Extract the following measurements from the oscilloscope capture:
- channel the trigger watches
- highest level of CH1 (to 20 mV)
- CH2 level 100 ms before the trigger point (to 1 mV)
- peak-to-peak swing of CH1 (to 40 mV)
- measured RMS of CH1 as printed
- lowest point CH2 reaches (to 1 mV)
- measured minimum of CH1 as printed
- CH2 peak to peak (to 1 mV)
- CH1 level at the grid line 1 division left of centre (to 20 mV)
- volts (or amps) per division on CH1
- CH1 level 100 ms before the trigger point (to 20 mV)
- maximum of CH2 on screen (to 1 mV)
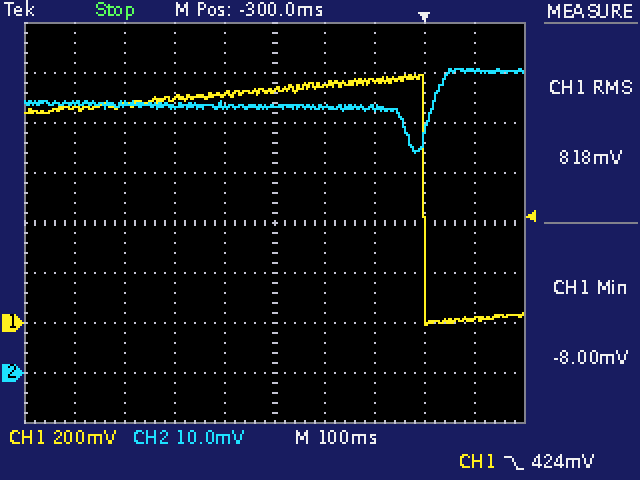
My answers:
CH1
1.00 V
53 mV
1.00 V
818 mV
44 mV
-8.00 mV
17 mV
920 mV
200 mV
960 mV
61 mV
